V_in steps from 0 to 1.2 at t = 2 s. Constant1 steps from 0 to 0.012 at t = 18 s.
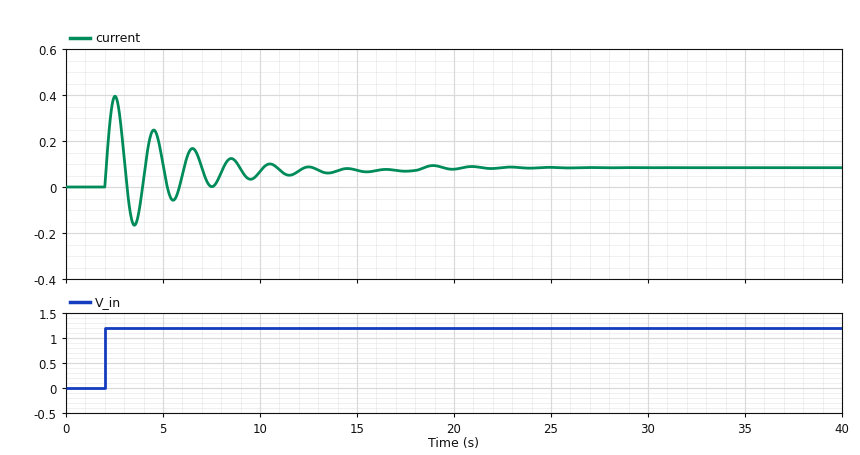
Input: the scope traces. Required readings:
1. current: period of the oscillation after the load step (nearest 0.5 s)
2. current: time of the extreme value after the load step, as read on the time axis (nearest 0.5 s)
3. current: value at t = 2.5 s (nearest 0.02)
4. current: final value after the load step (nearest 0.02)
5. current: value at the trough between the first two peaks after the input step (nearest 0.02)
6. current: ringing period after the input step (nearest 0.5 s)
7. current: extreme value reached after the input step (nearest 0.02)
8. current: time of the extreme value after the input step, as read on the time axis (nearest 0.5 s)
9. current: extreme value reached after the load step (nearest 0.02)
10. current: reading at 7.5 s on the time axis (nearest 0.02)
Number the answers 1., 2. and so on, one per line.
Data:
1. 2.0 s
2. 19.0 s
3. 0.40
4. 0.08
5. -0.16
6. 2.0 s
7. 0.40
8. 2.5 s
9. 0.10
10. 0.00
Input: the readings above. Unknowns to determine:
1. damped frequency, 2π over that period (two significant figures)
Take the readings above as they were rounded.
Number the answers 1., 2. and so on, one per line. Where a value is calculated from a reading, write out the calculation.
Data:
1. 2π / 2 = 3.1 rad/s
